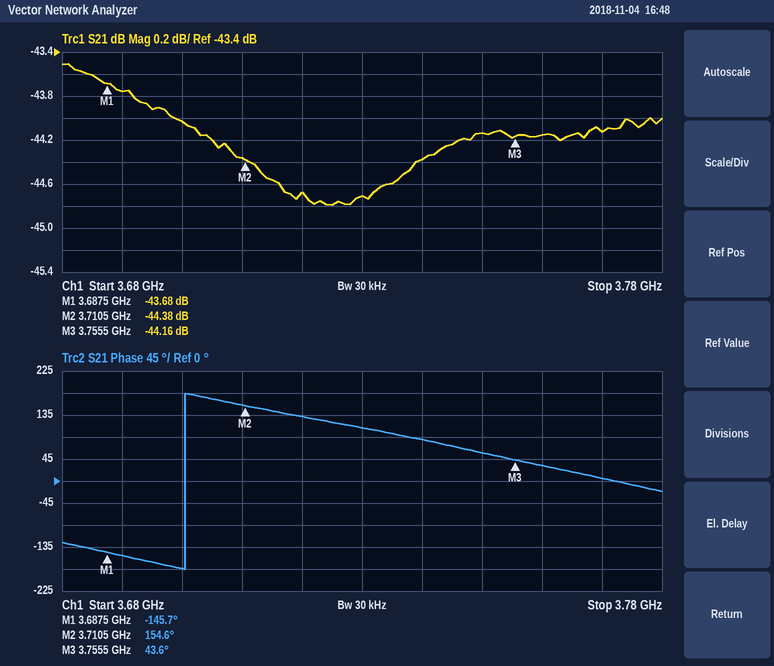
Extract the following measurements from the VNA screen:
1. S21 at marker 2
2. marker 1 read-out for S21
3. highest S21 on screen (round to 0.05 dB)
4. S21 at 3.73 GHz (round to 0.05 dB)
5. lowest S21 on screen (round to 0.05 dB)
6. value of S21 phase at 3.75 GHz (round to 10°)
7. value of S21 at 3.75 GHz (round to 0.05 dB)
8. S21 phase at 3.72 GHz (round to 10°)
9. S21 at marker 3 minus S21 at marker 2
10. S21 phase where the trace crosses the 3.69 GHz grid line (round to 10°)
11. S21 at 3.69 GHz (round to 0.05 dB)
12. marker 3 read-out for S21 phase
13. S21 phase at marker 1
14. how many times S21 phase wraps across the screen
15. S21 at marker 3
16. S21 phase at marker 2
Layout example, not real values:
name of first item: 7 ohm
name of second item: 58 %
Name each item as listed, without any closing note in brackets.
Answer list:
S21 at marker 2: -44.38 dB
marker 1 read-out for S21: -43.68 dB
highest S21 on screen: -43.50 dB
S21 at 3.73 GHz: -44.70 dB
lowest S21 on screen: -44.80 dB
value of S21 phase at 3.75 GHz: 60°
value of S21 at 3.75 GHz: -44.15 dB
S21 phase at 3.72 GHz: 130°
S21 at marker 3 minus S21 at marker 2: 0.22 dB
S21 phase where the trace crosses the 3.69 GHz grid line: -150°
S21 at 3.69 GHz: -43.75 dB
marker 3 read-out for S21 phase: 43.6°
S21 phase at marker 1: -145.7°
how many times S21 phase wraps across the screen: 1
S21 at marker 3: -44.16 dB
S21 phase at marker 2: 154.6°
